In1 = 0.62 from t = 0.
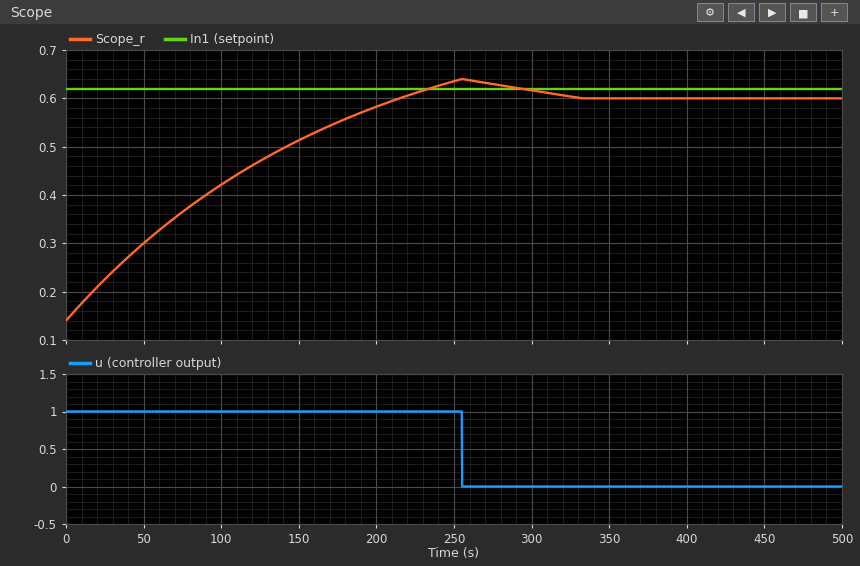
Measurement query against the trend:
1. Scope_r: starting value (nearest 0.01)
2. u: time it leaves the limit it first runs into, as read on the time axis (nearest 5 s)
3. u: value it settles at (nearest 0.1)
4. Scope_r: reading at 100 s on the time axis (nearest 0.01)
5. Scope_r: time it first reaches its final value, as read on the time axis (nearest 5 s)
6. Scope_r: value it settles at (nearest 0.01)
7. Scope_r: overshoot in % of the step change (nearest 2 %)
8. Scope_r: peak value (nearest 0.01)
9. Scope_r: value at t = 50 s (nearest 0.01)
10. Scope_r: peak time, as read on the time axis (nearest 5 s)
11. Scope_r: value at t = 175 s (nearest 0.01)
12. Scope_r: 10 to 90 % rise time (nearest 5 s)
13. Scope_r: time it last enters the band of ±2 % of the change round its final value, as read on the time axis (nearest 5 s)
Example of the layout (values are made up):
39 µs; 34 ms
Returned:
0.14; 255 s; 0.0; 0.42; 215 s; 0.60; 8 %; 0.64; 0.30; 255 s; 0.55; 165 s; 315 s
